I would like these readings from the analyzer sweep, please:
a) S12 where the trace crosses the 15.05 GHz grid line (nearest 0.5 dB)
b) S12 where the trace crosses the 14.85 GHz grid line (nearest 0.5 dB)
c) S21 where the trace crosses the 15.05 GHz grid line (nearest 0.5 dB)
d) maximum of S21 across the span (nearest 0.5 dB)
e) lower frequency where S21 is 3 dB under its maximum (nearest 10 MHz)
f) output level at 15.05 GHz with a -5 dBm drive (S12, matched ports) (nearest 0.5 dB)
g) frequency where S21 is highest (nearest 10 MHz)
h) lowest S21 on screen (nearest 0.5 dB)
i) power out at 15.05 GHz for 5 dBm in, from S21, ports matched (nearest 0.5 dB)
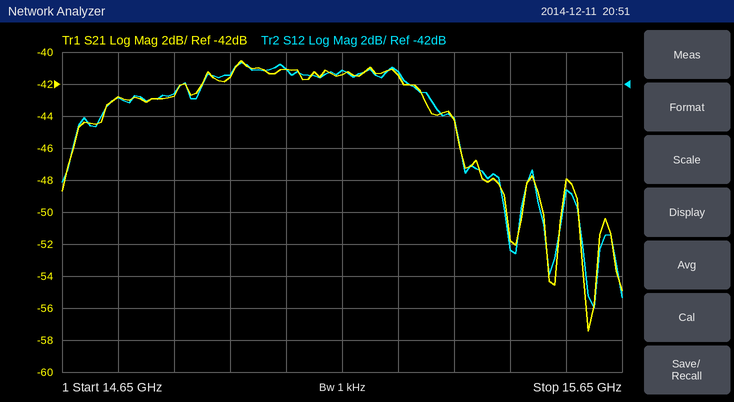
-41.0 dB
-42.5 dB
-41.0 dB
-40.5 dB
14.73 GHz
-46.0 dBm
14.97 GHz
-57.5 dB
-36.0 dBm
